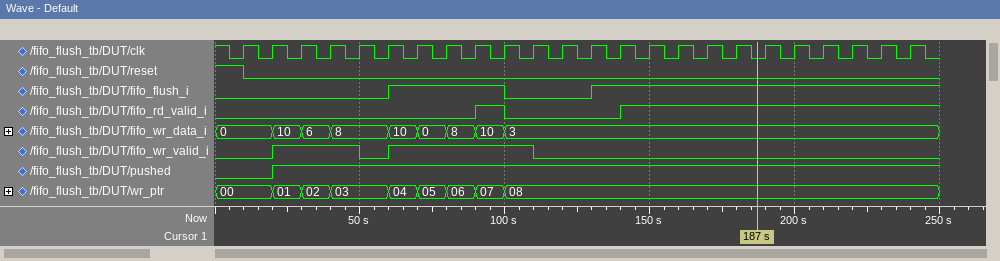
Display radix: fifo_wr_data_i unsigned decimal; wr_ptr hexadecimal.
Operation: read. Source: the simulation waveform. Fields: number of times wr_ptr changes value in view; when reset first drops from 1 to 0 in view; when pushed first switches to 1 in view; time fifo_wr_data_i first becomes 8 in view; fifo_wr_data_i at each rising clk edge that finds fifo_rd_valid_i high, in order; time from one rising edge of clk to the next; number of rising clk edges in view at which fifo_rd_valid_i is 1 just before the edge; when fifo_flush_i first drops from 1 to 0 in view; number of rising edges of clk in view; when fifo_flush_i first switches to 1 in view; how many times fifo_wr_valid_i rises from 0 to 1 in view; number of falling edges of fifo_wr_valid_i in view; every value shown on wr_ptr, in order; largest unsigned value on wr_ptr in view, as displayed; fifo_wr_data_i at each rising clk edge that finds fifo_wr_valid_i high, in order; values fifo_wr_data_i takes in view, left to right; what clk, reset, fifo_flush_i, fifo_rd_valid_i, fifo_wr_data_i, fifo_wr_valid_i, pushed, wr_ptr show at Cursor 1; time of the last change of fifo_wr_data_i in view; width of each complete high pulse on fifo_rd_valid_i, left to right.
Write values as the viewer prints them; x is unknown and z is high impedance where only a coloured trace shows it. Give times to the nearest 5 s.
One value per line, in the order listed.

8
10 s
20 s
40 s
10, 3, 3, 3, 3, 3, 3, 3, 3, 3, 3
10 s
11
100 s
24
60 s
2
2
00, 01, 02, 03, 04, 05, 06, 07, 08
08
10, 6, 8, 10, 0, 8, 10, 3
0, 10, 6, 8, 10, 0, 8, 10, 3
clk=0, reset=0, fifo_flush_i=1, fifo_rd_valid_i=1, fifo_wr_data_i=3, fifo_wr_valid_i=0, pushed=1, wr_ptr=08
100 s
10 s
